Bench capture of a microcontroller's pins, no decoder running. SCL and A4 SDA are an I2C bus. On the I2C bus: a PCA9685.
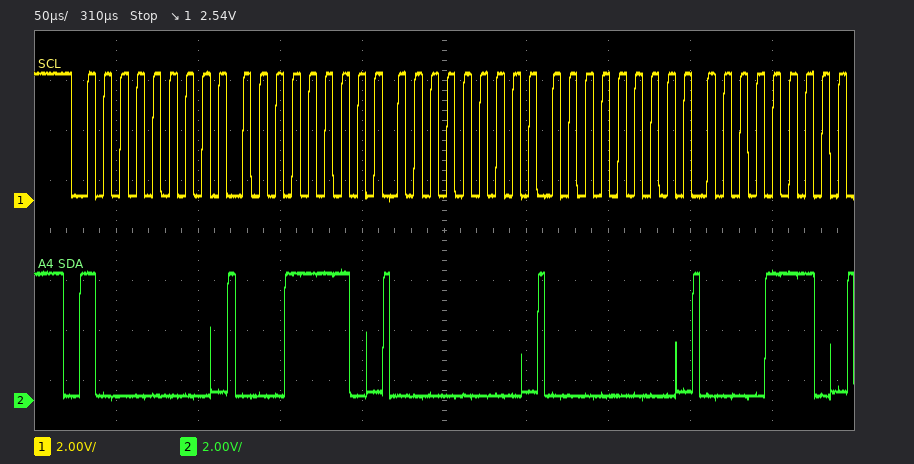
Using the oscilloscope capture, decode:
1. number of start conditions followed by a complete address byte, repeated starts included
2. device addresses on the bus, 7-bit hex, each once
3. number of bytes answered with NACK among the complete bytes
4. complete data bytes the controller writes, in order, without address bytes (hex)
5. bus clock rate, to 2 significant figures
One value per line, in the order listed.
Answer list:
1
0x40
0
1E 00 00 0E
100 kHz
